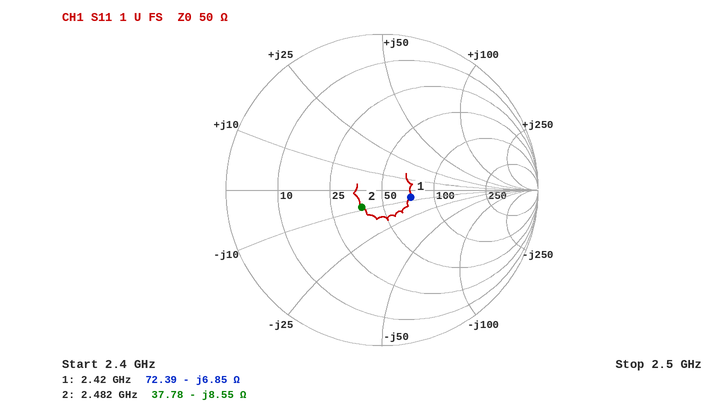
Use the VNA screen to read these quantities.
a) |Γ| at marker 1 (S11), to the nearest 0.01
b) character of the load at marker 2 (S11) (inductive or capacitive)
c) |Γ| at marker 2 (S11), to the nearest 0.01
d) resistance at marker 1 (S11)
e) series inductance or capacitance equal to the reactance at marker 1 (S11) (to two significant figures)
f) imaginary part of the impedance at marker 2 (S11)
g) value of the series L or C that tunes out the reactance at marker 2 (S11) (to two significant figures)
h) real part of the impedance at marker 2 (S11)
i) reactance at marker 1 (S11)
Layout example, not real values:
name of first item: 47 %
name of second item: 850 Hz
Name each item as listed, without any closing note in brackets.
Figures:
|Γ| at marker 1 (S11), to the nearest 0.01: 0.19
character of the load at marker 2 (S11): capacitive
|Γ| at marker 2 (S11), to the nearest 0.01: 0.17
resistance at marker 1: 72.39 Ω
series inductance or capacitance equal to the reactance at marker 1 (S11): 9.6 pF
imaginary part of the impedance at marker 2: -8.55 Ω
value of the series L or C that tunes out the reactance at marker 2 (S11): 550 pH
real part of the impedance at marker 2: 37.78 Ω
reactance at marker 1: -6.85 Ω
